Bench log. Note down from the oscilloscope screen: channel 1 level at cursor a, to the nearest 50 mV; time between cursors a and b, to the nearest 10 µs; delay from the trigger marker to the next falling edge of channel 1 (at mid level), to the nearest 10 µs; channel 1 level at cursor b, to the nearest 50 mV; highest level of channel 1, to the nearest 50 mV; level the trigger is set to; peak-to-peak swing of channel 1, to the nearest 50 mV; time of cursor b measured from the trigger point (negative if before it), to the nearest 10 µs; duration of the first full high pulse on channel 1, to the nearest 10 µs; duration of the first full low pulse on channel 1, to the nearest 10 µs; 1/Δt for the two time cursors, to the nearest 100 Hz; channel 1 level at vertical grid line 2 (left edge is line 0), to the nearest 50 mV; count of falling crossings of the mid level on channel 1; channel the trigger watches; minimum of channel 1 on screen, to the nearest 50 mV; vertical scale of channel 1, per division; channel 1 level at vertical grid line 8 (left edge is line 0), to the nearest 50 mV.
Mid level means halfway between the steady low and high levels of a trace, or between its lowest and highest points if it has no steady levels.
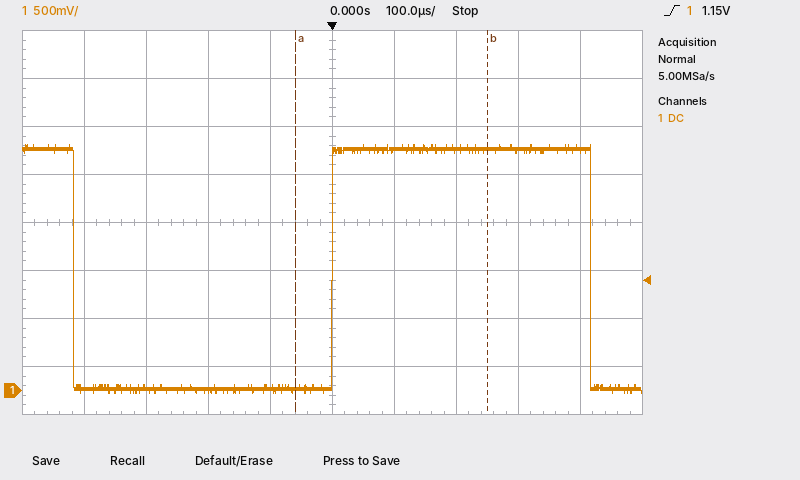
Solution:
0 mV
310 µs
420 µs
2.50 V
2.55 V
1.15 V
2.60 V
+250 µs
420 µs
420 µs
3.2 kHz
50 mV
2
channel 1
-50 mV
500 mV
2.50 V
